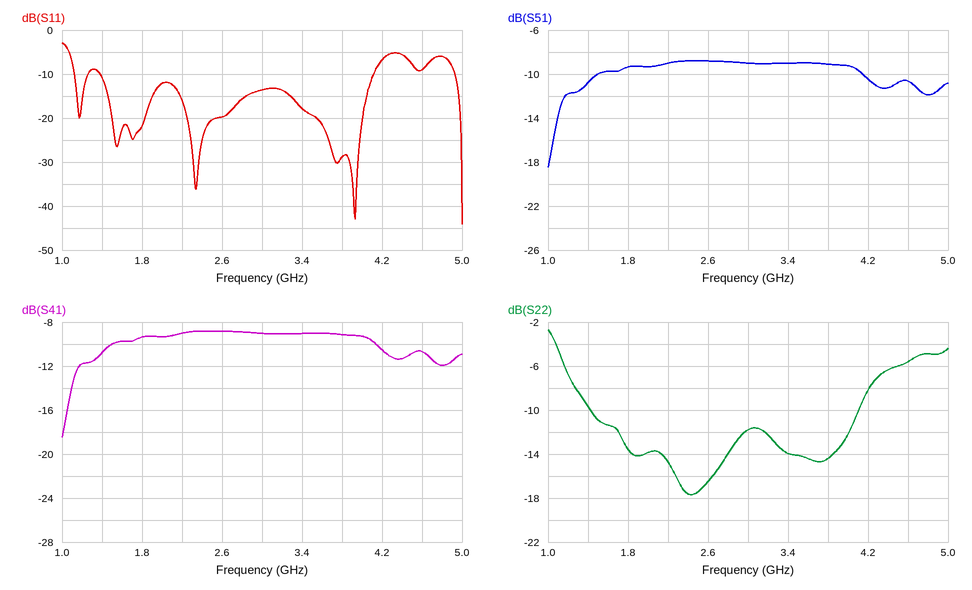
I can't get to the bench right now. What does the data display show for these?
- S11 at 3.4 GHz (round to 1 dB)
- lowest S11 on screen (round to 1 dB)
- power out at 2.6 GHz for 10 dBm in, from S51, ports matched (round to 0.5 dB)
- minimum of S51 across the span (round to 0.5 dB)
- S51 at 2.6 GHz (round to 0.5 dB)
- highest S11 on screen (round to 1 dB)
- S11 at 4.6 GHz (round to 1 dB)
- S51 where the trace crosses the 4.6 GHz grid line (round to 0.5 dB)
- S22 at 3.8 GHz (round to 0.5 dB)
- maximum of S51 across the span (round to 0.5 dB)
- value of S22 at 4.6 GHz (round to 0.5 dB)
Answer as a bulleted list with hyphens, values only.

- -18 dB
- -44 dB
- 1.0 dBm
- -18.5 dB
- -9.0 dB
- -3 dB
- -9 dB
- -10.5 dB
- -14.5 dB
- -9.0 dB
- -5.5 dB
